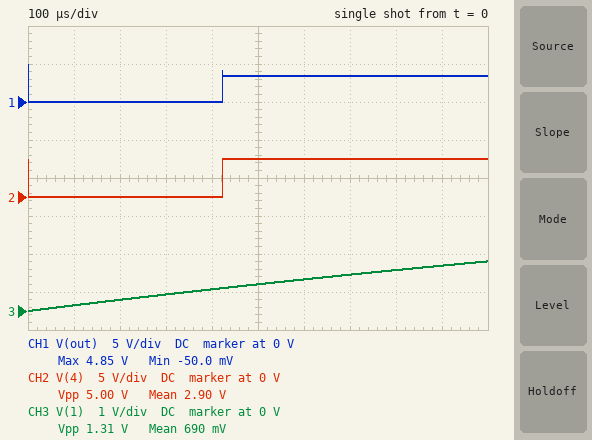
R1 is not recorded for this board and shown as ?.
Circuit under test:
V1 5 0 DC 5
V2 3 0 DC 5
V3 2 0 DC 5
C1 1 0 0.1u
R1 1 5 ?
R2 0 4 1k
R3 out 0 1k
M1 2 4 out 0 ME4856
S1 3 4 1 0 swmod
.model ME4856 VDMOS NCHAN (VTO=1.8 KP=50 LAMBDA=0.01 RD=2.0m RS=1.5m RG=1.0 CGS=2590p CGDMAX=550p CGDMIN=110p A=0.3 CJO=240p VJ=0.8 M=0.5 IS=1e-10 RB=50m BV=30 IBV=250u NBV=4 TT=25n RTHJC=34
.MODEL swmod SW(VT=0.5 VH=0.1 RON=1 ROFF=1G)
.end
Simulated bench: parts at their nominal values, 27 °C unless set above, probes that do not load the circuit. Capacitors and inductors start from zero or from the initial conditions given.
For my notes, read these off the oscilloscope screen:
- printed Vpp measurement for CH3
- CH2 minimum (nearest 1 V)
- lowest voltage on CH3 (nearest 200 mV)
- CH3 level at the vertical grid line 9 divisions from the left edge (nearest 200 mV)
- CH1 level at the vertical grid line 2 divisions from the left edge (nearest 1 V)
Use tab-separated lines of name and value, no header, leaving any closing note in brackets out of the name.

printed Vpp measurement for CH3	1.31 V
CH2 minimum	0 V
lowest voltage on CH3	0 V
CH3 level at the vertical grid line 9 divisions from the left edge	1.2 V
CH1 level at the vertical grid line 2 divisions from the left edge	0 V
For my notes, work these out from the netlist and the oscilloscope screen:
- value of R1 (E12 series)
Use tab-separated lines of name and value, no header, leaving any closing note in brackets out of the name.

value of R1	33 kΩ
